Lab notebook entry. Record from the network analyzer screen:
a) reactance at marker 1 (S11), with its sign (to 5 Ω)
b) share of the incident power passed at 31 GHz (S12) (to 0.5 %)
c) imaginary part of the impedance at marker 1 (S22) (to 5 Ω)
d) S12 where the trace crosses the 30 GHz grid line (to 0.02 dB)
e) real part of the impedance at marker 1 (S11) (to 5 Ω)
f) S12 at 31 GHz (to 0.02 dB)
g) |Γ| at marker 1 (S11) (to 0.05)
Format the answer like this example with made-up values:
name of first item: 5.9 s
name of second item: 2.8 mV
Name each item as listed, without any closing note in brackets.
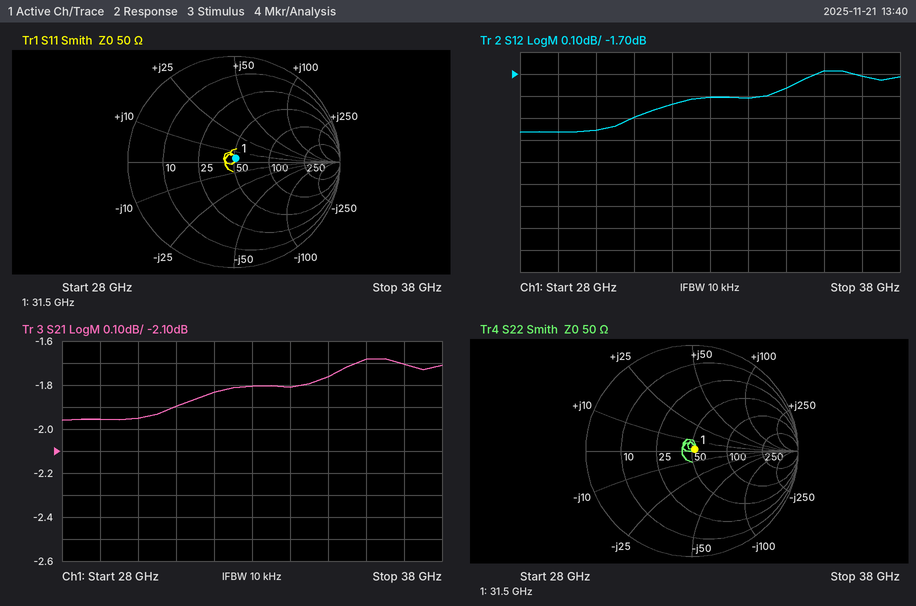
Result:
reactance at marker 1 (S11), with its sign: +5 Ω
share of the incident power passed at 31 GHz (S12): 64.5 %
imaginary part of the impedance at marker 1 (S22): 0 Ω
S12 where the trace crosses the 30 GHz grid line: -1.96 dB
real part of the impedance at marker 1 (S11): 50 Ω
S12 at 31 GHz: -1.90 dB
|Γ| at marker 1 (S11): 0.05
